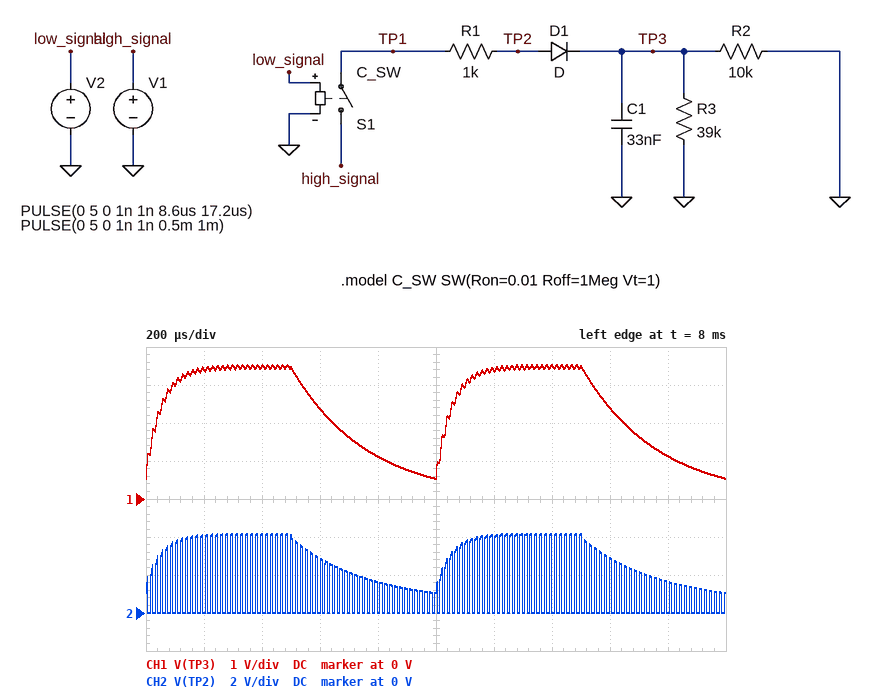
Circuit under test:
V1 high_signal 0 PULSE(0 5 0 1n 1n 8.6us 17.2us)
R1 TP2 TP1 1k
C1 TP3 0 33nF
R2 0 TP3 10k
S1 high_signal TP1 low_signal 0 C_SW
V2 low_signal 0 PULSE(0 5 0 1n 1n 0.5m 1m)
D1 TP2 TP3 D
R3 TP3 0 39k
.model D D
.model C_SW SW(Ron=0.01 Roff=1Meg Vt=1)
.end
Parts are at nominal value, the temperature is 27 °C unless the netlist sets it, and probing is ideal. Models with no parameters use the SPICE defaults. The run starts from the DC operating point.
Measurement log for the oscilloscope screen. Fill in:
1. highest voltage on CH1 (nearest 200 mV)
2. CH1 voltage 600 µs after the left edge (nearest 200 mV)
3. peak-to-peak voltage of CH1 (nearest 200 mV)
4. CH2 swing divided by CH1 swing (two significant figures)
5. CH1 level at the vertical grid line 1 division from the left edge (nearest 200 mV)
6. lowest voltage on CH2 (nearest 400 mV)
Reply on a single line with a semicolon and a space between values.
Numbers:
3.6 V; 2.4 V; 3.0 V; 1.4; 3.4 V; 0 V
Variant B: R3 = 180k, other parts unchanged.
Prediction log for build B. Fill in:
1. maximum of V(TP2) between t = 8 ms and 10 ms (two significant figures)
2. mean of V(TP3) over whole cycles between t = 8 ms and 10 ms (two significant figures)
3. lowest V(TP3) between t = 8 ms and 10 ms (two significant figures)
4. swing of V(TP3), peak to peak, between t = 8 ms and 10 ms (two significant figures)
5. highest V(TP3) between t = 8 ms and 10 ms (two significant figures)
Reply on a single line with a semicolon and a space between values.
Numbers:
4.3 V; 2.5 V; 730 mV; 2.9 V; 3.6 V
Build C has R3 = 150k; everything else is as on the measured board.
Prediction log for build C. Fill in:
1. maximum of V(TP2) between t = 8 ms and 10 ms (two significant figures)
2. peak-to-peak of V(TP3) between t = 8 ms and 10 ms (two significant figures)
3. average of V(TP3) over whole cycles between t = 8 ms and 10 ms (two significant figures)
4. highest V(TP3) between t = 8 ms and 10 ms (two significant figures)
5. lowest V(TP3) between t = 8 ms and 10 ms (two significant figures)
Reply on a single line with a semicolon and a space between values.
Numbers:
4.3 V; 2.9 V; 2.5 V; 3.6 V; 720 mV
